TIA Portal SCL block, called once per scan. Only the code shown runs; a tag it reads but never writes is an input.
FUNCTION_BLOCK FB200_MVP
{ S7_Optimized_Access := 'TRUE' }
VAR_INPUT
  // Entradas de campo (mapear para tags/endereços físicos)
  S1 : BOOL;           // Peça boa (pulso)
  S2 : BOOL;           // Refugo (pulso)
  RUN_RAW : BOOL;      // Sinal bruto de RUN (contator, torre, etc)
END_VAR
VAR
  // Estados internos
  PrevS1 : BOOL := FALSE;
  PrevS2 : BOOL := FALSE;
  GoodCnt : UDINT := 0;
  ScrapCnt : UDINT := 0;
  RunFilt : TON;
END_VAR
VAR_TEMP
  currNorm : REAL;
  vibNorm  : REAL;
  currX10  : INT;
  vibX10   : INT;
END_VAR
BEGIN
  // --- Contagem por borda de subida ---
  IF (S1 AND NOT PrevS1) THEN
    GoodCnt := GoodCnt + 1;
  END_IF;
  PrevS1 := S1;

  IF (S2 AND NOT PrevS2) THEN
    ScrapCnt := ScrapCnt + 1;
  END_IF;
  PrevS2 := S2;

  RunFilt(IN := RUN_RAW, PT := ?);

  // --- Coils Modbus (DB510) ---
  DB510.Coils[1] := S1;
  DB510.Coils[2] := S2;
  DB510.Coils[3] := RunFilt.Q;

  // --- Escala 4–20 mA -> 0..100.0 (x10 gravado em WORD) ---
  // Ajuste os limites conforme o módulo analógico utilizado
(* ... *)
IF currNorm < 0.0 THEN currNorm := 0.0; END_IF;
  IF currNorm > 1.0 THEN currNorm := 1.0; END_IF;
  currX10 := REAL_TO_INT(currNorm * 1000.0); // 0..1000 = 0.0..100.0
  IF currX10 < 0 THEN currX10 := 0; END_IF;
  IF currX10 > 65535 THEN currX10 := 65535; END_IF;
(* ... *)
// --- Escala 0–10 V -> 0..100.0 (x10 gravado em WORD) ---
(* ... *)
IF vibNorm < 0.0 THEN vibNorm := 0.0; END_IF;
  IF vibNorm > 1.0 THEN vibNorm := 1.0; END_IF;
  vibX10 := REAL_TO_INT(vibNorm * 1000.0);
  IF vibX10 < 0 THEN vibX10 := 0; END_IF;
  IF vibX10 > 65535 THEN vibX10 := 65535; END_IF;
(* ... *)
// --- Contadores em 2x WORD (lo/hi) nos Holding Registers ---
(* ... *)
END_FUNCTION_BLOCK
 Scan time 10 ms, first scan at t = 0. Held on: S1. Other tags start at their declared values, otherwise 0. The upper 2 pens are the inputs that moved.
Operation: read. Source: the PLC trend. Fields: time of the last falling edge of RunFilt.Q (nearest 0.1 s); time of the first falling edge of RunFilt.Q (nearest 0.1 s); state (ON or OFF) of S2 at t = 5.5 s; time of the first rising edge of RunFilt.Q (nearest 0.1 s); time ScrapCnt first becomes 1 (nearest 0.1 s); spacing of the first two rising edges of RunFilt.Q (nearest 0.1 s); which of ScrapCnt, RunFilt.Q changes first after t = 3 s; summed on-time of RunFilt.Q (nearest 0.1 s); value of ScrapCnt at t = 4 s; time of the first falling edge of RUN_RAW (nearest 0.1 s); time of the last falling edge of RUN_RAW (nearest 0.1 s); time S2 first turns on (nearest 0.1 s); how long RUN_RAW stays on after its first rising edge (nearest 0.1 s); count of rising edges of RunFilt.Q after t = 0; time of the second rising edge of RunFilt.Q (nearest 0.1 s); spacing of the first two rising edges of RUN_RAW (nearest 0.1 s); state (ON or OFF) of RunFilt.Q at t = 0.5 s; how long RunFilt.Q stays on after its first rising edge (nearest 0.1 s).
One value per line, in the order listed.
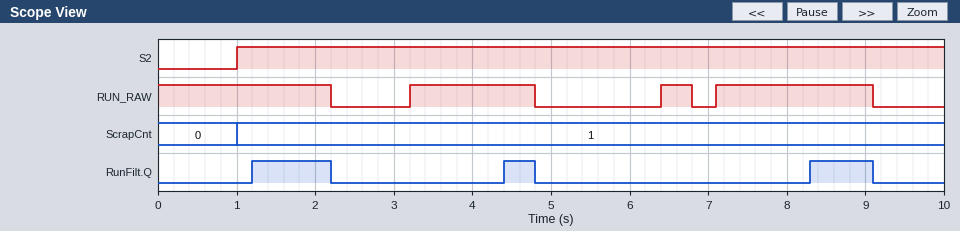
9.1 s
2.2 s
ON
1.2 s
1.0 s
3.2 s
RunFilt.Q
2.2 s
1
2.2 s
9.1 s
1.0 s
1.6 s
3
4.4 s
3.2 s
OFF
1.0 s
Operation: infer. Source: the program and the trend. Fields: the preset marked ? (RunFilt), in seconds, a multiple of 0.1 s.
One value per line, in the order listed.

1.2 s
